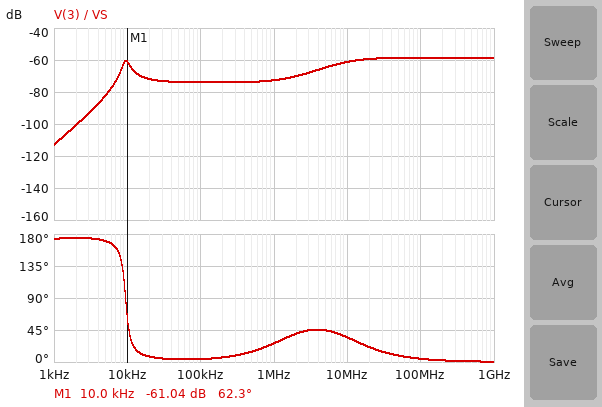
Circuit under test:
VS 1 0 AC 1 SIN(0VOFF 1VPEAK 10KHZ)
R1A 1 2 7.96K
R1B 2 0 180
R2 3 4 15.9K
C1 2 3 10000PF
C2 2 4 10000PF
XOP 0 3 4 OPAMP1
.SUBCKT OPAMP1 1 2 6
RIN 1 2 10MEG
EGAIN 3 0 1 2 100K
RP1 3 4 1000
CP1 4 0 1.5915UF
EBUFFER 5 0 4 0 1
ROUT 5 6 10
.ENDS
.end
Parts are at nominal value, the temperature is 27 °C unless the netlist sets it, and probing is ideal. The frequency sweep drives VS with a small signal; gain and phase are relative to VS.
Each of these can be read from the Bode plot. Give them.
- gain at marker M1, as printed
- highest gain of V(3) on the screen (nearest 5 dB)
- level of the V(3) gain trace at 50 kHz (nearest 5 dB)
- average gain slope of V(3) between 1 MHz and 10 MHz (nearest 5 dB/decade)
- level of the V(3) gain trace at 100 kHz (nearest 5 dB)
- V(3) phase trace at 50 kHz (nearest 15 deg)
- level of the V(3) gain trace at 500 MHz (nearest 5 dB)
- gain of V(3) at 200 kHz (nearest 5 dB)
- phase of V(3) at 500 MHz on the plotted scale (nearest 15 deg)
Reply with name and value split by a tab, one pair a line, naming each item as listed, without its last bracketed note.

gain at marker M1, as printed	-61.04 dB
highest gain of V(3) on the screen	-60 dB
level of the V(3) gain trace at 50 kHz	-75 dB
average gain slope of V(3) between 1 MHz and 10 MHz	10 dB/decade
level of the V(3) gain trace at 100 kHz	-75 dB
V(3) phase trace at 50 kHz	0 deg
level of the V(3) gain trace at 500 MHz	-60 dB
gain of V(3) at 200 kHz	-75 dB
phase of V(3) at 500 MHz on the plotted scale	0 deg
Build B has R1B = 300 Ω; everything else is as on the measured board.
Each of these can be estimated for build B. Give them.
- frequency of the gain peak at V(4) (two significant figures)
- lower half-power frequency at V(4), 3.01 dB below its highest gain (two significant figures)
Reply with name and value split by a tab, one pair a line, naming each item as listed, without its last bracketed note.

frequency of the gain peak at V(4)	7.4 kHz
lower half-power frequency at V(4), 3.01 dB below its highest gain	6.5 kHz
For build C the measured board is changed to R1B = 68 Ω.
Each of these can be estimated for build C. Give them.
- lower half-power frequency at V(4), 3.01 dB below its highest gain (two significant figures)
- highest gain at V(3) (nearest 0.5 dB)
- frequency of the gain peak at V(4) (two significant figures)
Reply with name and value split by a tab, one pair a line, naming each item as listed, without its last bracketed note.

lower half-power frequency at V(4), 3.01 dB below its highest gain	14 kHz
highest gain at V(3)	-56.5 dB
frequency of the gain peak at V(4)	15 kHz
